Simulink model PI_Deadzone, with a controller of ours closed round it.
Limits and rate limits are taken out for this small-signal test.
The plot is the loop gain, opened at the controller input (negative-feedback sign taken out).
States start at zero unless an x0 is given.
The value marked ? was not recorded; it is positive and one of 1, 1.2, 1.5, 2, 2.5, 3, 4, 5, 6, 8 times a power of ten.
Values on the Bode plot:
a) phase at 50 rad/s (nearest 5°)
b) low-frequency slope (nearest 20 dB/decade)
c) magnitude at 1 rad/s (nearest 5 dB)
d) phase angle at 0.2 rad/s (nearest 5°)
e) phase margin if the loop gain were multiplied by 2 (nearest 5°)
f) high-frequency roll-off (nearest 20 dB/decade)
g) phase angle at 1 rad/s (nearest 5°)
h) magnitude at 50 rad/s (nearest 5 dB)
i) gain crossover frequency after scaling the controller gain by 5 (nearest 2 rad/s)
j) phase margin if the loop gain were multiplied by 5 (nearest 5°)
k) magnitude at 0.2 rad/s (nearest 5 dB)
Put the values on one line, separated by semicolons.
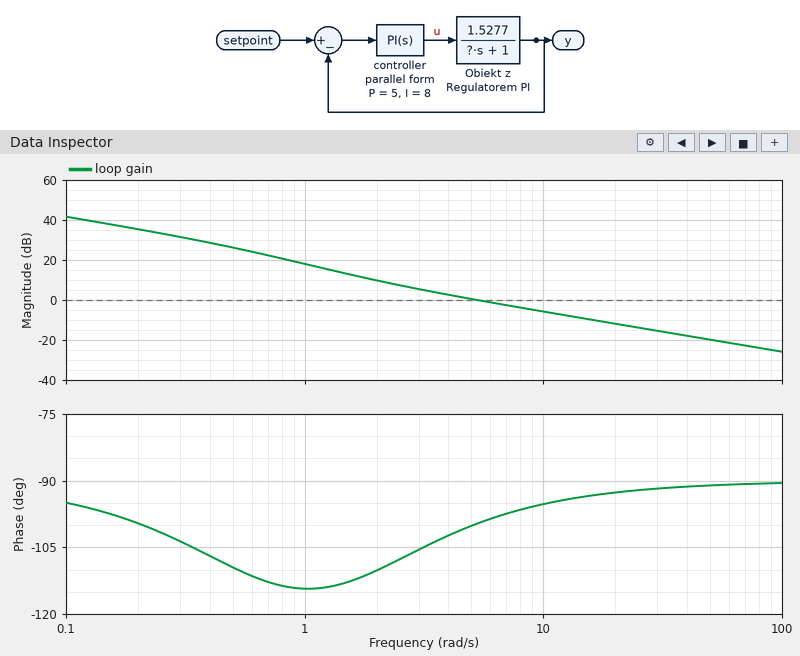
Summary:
-90°; -20 dB/decade; 20 dB; -100°; 85°; -20 dB/decade; -115°; -20 dB; 26 rad/s; 90°; 35 dB
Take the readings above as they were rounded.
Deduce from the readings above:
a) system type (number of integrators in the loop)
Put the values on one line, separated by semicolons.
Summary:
1
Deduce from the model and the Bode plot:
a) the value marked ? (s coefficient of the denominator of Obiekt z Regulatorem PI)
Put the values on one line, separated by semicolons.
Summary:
1.5
